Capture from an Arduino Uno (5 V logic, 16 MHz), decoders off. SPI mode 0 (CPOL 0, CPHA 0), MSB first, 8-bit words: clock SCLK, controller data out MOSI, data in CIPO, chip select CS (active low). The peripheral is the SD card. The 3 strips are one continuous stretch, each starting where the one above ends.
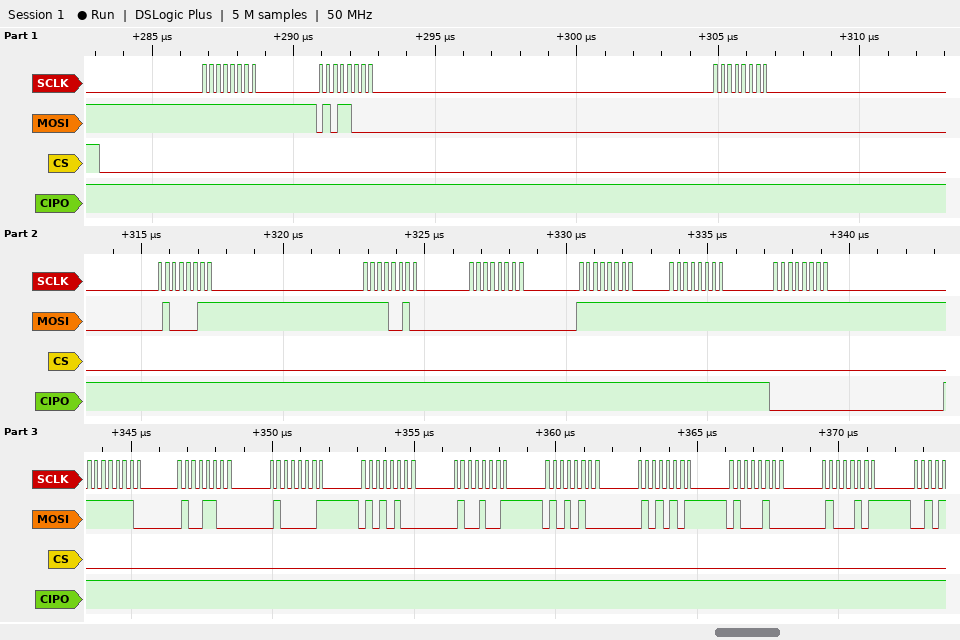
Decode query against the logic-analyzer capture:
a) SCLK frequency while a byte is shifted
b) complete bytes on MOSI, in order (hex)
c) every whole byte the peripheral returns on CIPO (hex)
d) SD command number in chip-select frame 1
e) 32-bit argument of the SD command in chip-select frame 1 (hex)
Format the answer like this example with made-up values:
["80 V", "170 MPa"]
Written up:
["4 MHz", "0xFF 0x58 0x00 0x43 0xF2 0x00 0xFF 0xFF 0xFF 0xFE 0x4C 0x41 0x54 0x49 0x54 0x55 0x44 0x45", "0xFF 0xFF 0xFF 0xFF 0xFF 0xFF 0xFF 0xFF 0x00 0xFF 0xFF 0xFF 0xFF 0xFF 0xFF 0xFF 0xFF 0xFF", "CMD24", "0x0043F200"]
